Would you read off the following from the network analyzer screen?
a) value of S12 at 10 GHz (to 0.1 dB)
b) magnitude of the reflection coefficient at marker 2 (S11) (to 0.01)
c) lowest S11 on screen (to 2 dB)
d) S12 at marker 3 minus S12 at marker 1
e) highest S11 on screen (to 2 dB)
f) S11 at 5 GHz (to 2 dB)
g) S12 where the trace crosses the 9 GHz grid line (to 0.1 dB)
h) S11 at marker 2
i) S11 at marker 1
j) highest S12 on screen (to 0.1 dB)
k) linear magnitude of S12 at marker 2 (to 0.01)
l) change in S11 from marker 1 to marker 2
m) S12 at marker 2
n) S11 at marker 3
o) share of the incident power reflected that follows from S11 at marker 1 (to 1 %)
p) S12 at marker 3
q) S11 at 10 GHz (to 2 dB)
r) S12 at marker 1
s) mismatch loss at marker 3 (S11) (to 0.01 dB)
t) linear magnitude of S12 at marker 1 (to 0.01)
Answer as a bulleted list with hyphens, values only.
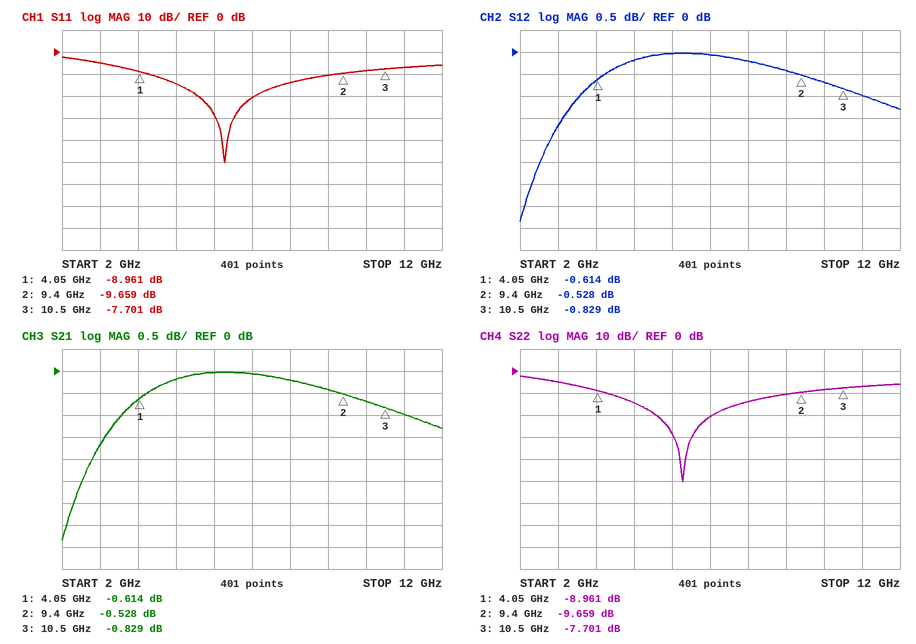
- -0.7 dB
- 0.33
- -50 dB
- -0.215 dB
- -2 dB
- -14 dB
- -0.4 dB
- -9.659 dB
- -8.961 dB
- 0.0 dB
- 0.94
- -0.698 dB
- -0.528 dB
- -7.701 dB
- 13 %
- -0.829 dB
- -8 dB
- -0.614 dB
- 0.81 dB
- 0.93
